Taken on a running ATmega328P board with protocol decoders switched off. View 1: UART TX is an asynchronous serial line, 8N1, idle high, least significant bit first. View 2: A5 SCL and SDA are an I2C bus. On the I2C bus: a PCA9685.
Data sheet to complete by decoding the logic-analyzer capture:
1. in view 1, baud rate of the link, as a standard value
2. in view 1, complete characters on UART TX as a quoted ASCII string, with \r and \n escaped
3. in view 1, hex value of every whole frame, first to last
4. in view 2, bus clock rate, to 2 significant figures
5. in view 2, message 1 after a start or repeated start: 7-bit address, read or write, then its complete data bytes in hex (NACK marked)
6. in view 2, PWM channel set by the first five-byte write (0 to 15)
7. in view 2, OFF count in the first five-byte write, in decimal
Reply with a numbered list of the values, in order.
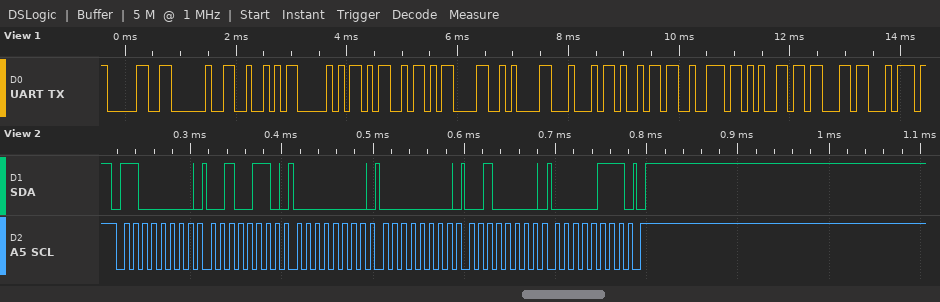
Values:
1. 9600 baud
2. "0 RPM\r\nDirect"
3. 30 20 52 50 4D 0D 0A 44 69 72 65 63 74
4. 100 kHz
5. 0x60 write: 26 00 00 20 07
6. 8
7. 1824
